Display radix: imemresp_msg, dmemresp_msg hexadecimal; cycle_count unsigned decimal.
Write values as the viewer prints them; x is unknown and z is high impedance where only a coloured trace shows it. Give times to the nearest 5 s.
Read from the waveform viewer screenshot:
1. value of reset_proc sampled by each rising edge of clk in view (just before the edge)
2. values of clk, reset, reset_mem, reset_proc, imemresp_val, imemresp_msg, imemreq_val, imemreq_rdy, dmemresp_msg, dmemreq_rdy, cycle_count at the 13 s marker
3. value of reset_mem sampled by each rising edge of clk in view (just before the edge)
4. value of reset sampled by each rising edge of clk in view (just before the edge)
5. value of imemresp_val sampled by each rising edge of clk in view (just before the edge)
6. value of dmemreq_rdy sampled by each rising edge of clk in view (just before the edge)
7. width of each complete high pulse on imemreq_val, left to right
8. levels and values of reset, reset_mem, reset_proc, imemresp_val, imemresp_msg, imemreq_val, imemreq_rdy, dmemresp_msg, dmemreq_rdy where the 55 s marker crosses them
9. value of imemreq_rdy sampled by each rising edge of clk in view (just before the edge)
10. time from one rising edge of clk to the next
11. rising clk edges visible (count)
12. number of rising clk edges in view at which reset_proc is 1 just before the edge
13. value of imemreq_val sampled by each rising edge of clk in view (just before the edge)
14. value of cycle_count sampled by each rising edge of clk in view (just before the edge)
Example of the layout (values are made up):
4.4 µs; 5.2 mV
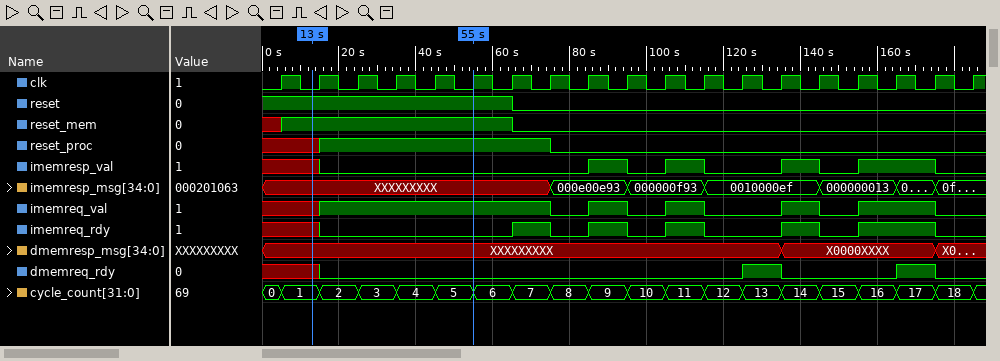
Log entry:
x x 1 1 1 1 1 1 0 0 0 0 0 0 0 0 0 0 0; clk=0, reset=1, reset_mem=1, reset_proc=x, imemresp_val=x, imemresp_msg=XXXXXXXXX, imemreq_val=x, imemreq_rdy=x, dmemresp_msg=XXXXXXXXX, dmemreq_rdy=x, cycle_count=1; x 1 1 1 1 1 1 0 0 0 0 0 0 0 0 0 0 0 0; 1 1 1 1 1 1 1 0 0 0 0 0 0 0 0 0 0 0 0; x x 0 0 0 0 0 0 0 1 0 1 0 0 1 0 1 1 0; x x 0 0 0 0 0 0 0 0 0 0 0 1 0 0 0 1 0; 10 s, 10 s, 10 s, 20 s; reset=1, reset_mem=1, reset_proc=1, imemresp_val=0, imemresp_msg=XXXXXXXXX, imemreq_val=1, imemreq_rdy=0, dmemresp_msg=XXXXXXXXX, dmemreq_rdy=0; x x 0 0 0 0 0 1 0 1 0 1 0 0 1 0 1 1 0; 10 s; 19; 6; x x 1 1 1 1 1 1 0 1 0 1 0 0 1 0 1 1 0; 0, 1, 2, 3, 4, 5, 6, 7, 8, 9, 10, 11, 12, 13, 14, 15, 16, 17, 18
